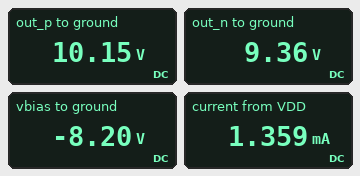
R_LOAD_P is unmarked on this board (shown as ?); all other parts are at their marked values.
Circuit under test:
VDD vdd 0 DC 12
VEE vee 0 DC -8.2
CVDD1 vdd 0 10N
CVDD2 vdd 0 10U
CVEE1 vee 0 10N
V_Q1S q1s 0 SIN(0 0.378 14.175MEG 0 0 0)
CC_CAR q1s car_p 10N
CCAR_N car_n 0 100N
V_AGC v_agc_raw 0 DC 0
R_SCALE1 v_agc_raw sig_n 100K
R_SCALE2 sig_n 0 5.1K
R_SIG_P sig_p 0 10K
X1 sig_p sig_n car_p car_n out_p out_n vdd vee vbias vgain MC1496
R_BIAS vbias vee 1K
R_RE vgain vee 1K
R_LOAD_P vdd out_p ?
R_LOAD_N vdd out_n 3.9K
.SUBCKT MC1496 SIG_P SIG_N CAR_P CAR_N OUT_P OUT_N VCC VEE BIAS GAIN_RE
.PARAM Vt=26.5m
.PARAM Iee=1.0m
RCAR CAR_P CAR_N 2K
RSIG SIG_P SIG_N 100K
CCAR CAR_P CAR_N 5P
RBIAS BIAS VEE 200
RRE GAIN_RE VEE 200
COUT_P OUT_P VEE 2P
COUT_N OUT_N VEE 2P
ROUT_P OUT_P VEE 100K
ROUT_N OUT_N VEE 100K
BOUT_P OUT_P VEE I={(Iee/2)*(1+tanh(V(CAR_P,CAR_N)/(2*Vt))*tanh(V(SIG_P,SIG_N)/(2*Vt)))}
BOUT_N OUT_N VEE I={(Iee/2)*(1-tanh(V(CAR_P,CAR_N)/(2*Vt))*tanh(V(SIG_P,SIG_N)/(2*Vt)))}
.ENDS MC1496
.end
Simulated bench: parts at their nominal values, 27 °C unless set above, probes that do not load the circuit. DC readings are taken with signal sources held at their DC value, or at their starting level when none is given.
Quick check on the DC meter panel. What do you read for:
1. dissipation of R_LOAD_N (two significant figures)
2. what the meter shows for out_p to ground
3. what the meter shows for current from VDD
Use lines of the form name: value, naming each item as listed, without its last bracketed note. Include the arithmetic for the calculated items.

dissipation of R_LOAD_N: (12 V - 9.36 V)^2 / 3.9 kΩ = 1.8 mW
what the meter shows for out_p to ground: 10.15 V
what the meter shows for current from VDD: 1.359 mA
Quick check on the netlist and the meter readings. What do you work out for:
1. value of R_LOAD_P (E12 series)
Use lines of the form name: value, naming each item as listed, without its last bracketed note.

value of R_LOAD_P: 2.7 kΩ
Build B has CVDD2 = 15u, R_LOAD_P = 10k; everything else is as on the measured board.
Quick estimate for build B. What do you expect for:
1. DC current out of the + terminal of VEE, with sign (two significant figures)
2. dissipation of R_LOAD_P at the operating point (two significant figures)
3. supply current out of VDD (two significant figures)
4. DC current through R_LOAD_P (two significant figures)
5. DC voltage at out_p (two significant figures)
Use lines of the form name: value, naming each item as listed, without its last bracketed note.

DC current out of the + terminal of VEE, with sign: -1.3 mA
dissipation of R_LOAD_P at the operating point: 4.1 mW
supply current out of VDD: 1.3 mA
DC current through R_LOAD_P: 640 µA
DC voltage at out_p: 5.6 V
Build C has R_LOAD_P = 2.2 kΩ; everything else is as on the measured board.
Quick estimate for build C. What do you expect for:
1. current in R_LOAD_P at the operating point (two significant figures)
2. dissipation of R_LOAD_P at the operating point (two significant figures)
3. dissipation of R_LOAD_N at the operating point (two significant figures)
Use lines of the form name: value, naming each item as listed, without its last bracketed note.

current in R_LOAD_P at the operating point: 690 µA
dissipation of R_LOAD_P at the operating point: 1.0 mW
dissipation of R_LOAD_N at the operating point: 1.8 mW
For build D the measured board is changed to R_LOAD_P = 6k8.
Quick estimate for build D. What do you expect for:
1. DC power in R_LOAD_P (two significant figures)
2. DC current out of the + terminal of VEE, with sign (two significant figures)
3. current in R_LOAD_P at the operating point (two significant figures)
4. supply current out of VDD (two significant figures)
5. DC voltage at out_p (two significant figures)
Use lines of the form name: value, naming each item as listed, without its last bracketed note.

DC power in R_LOAD_P: 2.9 mW
DC current out of the + terminal of VEE, with sign: -1.3 mA
current in R_LOAD_P at the operating point: 660 µA
supply current out of VDD: 1.3 mA
DC voltage at out_p: 7.5 V
